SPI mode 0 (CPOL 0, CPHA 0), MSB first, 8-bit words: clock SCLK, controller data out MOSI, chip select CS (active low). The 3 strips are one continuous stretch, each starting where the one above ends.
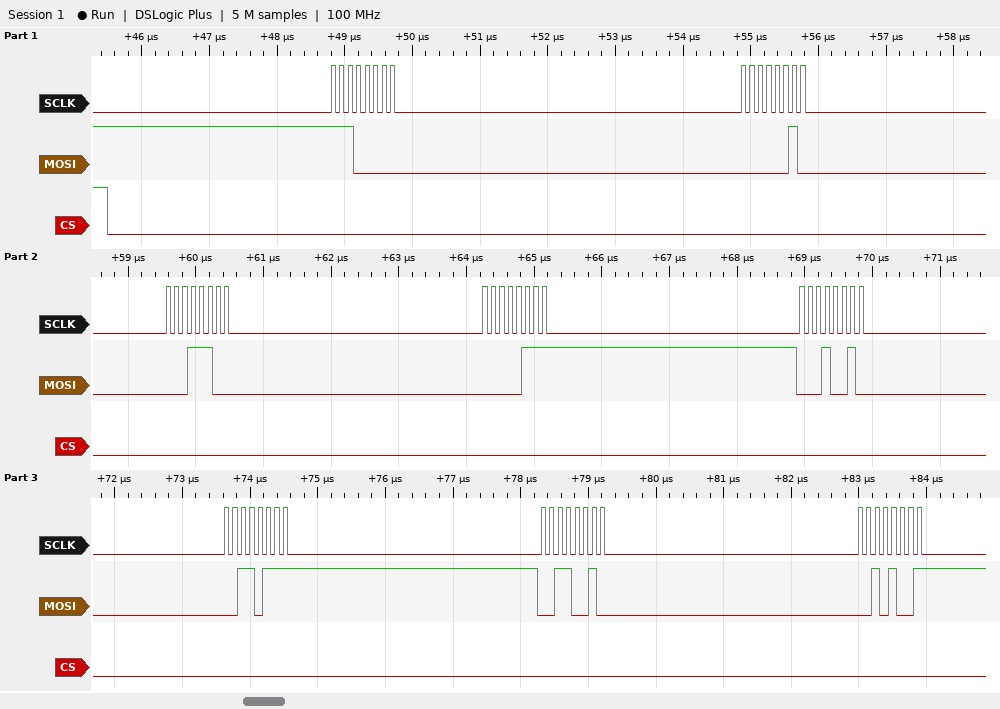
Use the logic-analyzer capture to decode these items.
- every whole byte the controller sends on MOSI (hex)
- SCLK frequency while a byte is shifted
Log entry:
0xE0 0x02 0x1C 0x07 0x12 0x37 0x32 0x29
8 MHz
